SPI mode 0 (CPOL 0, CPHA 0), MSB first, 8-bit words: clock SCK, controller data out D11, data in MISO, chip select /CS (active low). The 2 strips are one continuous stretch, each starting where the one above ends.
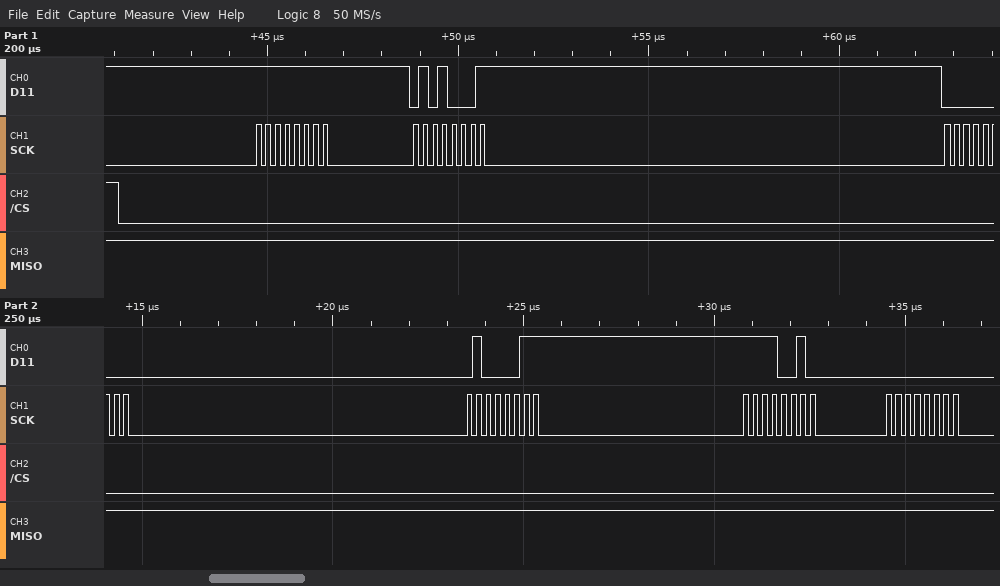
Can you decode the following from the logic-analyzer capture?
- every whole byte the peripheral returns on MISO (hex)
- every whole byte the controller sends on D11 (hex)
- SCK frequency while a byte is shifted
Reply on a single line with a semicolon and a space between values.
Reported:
FF FF FF FF FF FF; FF 51 00 43 F2 00; 4 MHz
